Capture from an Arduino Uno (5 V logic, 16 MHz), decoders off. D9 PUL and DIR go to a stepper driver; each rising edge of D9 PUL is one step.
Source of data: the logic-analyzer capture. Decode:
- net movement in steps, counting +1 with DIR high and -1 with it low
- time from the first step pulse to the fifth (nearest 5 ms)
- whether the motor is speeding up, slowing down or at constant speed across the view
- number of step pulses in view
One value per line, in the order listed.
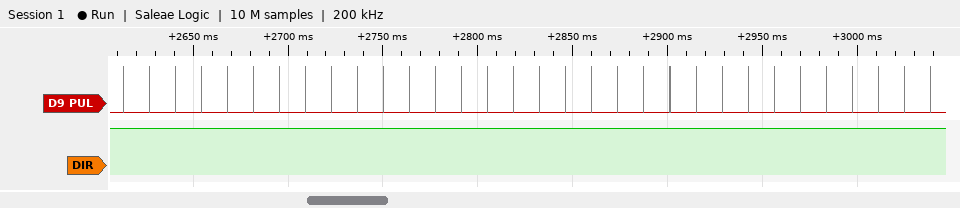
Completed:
+32
55 ms
constant speed
32
